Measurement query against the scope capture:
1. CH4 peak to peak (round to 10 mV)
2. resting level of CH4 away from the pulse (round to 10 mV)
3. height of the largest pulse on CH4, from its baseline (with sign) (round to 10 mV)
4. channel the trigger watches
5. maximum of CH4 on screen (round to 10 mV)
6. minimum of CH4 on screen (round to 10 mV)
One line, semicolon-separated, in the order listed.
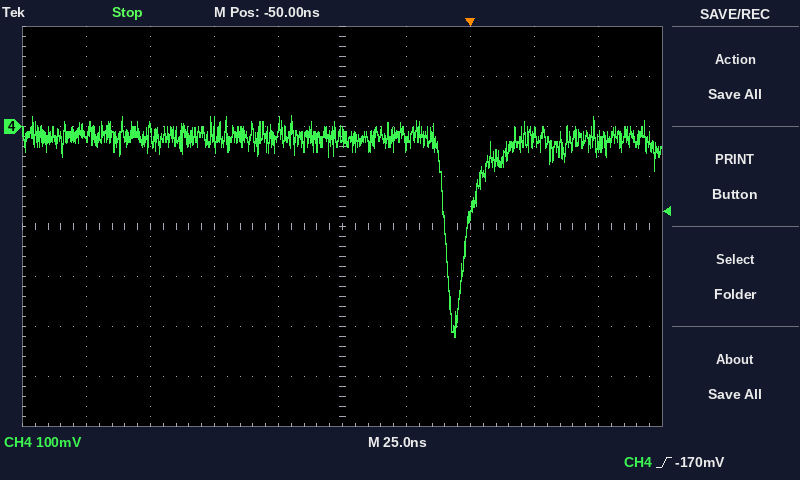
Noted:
440 mV; -20 mV; -400 mV; CH4; 20 mV; -420 mV
